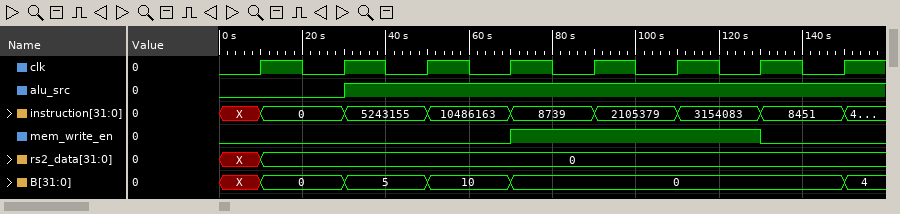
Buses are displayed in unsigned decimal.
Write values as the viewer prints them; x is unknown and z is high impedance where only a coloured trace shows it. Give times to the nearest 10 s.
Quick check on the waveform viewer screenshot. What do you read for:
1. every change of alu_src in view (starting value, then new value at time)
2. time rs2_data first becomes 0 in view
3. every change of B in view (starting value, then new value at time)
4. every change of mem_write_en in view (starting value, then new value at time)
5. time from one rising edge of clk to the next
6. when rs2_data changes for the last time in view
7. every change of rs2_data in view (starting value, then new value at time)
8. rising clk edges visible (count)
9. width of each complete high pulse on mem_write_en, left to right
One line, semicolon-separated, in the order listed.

0, 1 at 30 s; 10 s; X, 0 at 10 s, 5 at 30 s, 10 at 50 s, 0 at 70 s, 4 at 150 s; 0, 1 at 70 s, 0 at 130 s; 20 s; 10 s; X, 0 at 10 s; 8; 60 s
